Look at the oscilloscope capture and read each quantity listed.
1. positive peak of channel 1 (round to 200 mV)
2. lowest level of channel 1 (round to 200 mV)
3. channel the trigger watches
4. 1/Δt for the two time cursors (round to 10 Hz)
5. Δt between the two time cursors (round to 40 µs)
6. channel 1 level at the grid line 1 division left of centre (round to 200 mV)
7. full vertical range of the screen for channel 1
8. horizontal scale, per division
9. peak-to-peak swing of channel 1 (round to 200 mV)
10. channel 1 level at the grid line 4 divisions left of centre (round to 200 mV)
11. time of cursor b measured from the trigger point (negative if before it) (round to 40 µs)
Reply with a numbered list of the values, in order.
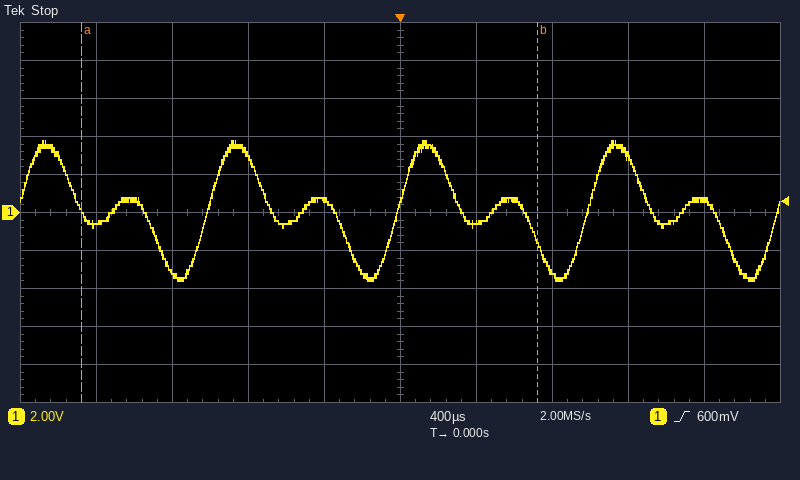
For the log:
1. 3.8 V
2. -3.6 V
3. channel 1
4. 420 Hz
5. 2.40 ms
6. 600 mV
7. 20 V
8. 400 µs
9. 7.4 V
10. -600 mV
11. +720 µs
